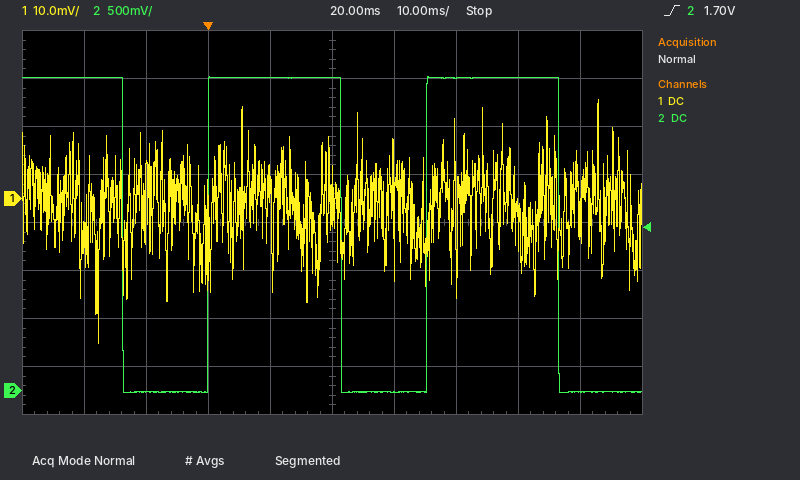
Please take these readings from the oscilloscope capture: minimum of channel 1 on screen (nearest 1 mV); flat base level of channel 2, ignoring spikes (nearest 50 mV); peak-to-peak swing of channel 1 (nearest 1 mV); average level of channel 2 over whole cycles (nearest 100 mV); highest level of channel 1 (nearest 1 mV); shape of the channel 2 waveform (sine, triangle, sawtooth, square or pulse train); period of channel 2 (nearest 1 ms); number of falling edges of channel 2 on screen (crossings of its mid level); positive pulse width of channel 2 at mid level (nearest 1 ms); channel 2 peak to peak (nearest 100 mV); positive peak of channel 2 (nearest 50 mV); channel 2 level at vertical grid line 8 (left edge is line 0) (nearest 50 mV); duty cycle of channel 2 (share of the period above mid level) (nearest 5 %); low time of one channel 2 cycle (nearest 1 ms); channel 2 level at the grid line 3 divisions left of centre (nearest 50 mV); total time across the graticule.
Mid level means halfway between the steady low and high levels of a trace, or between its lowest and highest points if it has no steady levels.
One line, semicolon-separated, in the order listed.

-30 mV; 0 mV; 51 mV; 2.0 V; 21 mV; pulse train; 35 ms; 3; 21 ms; 3.30 V; 3.25 V; 3.25 V; 60 %; 14 ms; 0 mV; 100 ms
